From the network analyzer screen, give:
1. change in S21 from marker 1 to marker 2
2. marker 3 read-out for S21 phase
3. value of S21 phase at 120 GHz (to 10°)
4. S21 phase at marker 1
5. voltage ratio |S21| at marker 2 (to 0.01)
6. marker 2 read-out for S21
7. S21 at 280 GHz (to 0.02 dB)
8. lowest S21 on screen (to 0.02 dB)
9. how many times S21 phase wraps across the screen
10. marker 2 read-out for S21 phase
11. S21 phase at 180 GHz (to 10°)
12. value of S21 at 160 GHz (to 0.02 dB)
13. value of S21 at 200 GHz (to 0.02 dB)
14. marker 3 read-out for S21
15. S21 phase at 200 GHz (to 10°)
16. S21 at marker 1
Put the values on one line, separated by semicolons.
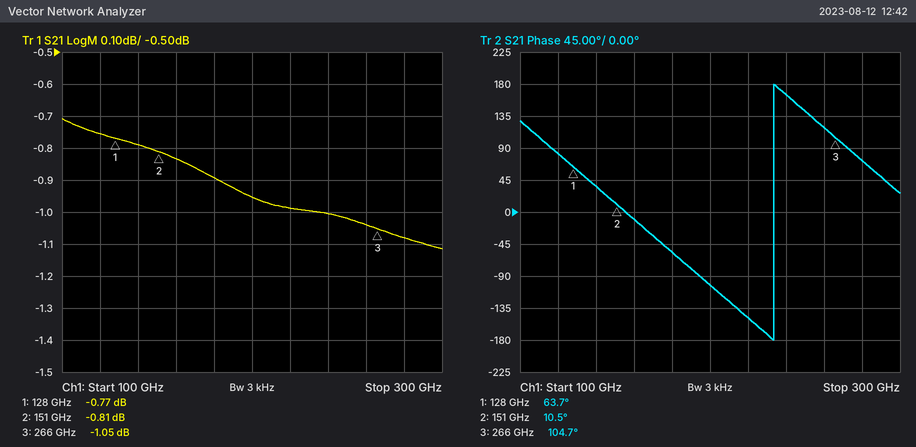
-0.04 dB; 104.7°; 80°; 63.7°; 0.91; -0.81 dB; -1.08 dB; -1.12 dB; 1; 10.5°; -60°; -0.84 dB; -0.96 dB; -1.05 dB; -100°; -0.77 dB
